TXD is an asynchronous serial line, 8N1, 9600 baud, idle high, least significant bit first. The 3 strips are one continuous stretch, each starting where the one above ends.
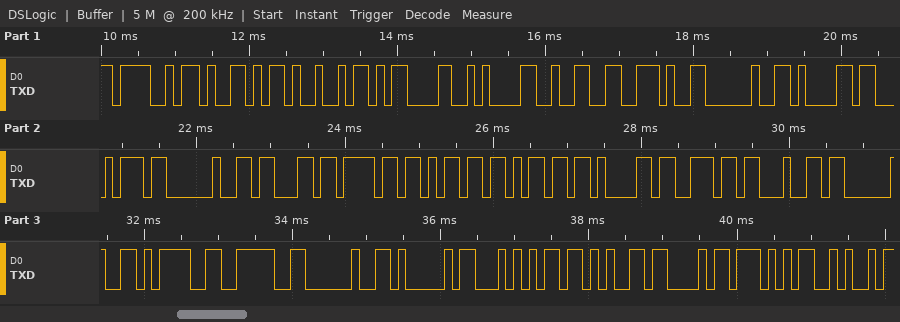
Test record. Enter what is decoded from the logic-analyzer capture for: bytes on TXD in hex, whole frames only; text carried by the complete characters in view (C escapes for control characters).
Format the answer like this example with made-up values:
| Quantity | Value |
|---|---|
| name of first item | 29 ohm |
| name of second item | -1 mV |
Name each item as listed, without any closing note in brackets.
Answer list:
| Quantity | Value |
|---|---|
| bytes on TXD in hex, whole frames only | 4F 59 49 0D 0A 32 2E 20 61 74 20 63 6F 6D 6D 61 6E 64 20 3D 3E 20 41 54 2B 43 57 4A |
| text carried by the complete characters in view | "OYI\r\n2. at command => AT+CWJ" |
